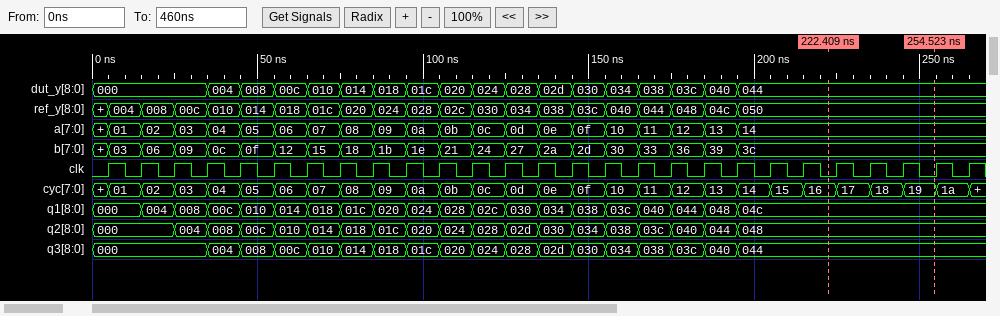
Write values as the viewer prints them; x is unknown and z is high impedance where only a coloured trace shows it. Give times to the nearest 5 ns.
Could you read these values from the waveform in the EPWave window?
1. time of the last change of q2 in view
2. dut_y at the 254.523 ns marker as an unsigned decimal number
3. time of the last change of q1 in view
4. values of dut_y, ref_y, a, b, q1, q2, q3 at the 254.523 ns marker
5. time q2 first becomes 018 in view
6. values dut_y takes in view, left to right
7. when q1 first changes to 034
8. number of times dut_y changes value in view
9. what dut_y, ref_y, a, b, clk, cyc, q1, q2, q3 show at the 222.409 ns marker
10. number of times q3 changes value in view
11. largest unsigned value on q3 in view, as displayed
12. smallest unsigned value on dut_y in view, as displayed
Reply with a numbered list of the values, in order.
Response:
1. 195 ns
2. 68
3. 195 ns
4. dut_y=044, ref_y=050, a=14, b=3c, q1=04c, q2=048, q3=044
5. 75 ns
6. 000, 004, 008, 00c, 010, 014, 018, 01c, 020, 024, 028, 02d, 030, 034, 038, 03c, 040, 044
7. 135 ns
8. 17
9. dut_y=044, ref_y=050, a=14, b=3c, clk=0, cyc=16, q1=04c, q2=048, q3=044
10. 17
11. 044
12. 000
